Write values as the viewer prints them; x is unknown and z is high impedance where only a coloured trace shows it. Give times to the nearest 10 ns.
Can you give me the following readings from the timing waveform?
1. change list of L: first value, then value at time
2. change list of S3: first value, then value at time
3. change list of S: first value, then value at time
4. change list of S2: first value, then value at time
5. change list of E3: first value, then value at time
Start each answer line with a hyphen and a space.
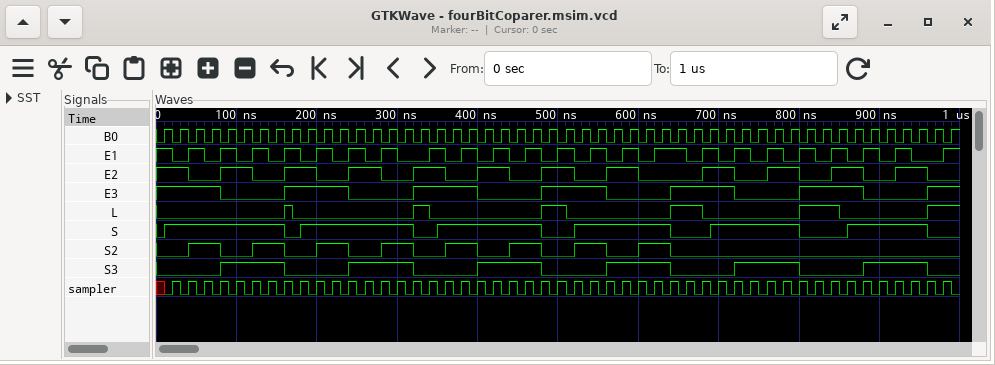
- 0, 1 at 160 ns, 0 at 170 ns, 1 at 320 ns, 0 at 340 ns, 1 at 480 ns, 0 at 510 ns, 1 at 640 ns, 0 at 680 ns, 1 at 800 ns, 0 at 850 ns, 1 at 960 ns
- 0, 1 at 80 ns, 0 at 160 ns, 1 at 240 ns, 0 at 320 ns, 1 at 400 ns, 0 at 480 ns, 1 at 560 ns, 0 at 640 ns, 1 at 720 ns, 0 at 800 ns, 1 at 880 ns, 0 at 960 ns
- 0, 1 at 10 ns, 0 at 160 ns, 1 at 180 ns, 0 at 320 ns, 1 at 350 ns, 0 at 480 ns, 1 at 520 ns, 0 at 640 ns, 1 at 690 ns, 0 at 800 ns, 1 at 860 ns, 0 at 960 ns
- 0, 1 at 40 ns, 0 at 80 ns, 1 at 120 ns, 0 at 160 ns, 1 at 200 ns, 0 at 240 ns, 1 at 280 ns, 0 at 320 ns, 1 at 360 ns, 0 at 400 ns, 1 at 440 ns, 0 at 480 ns, 1 at 520 ns, 0 at 560 ns, 1 at 600 ns, 0 at 640 ns
- 1, 0 at 80 ns, 1 at 160 ns, 0 at 240 ns, 1 at 320 ns, 0 at 400 ns, 1 at 480 ns, 0 at 560 ns, 1 at 640 ns, 0 at 720 ns, 1 at 800 ns, 0 at 880 ns, 1 at 960 ns
